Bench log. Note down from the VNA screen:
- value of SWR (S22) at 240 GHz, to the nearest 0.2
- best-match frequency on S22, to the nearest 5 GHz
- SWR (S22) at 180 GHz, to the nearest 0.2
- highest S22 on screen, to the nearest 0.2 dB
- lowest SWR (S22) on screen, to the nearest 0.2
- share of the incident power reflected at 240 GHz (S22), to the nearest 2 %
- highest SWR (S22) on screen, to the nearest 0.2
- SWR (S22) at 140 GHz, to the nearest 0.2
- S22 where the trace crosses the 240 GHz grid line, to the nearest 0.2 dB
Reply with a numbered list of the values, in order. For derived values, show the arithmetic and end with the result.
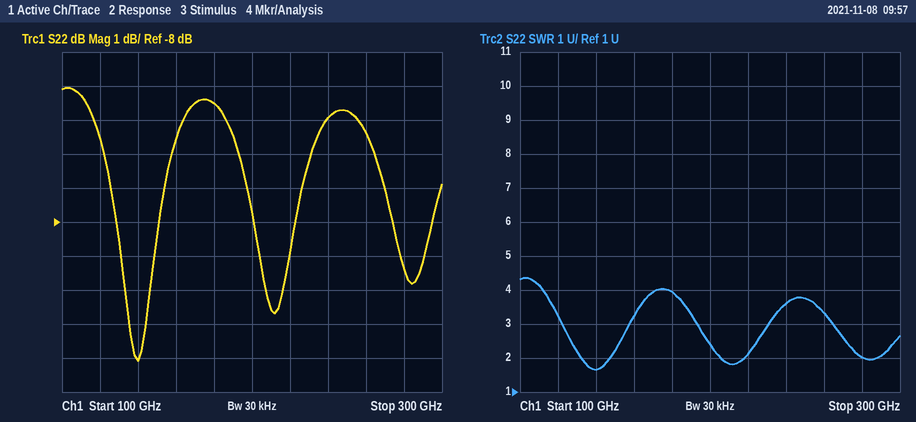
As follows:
1. 3.6
2. 140 GHz
3. 4.0
4. -4.0 dB
5. 1.6
6. 10^(-5/10) ≈ 32 %
7. 4.4
8. 1.6
9. -5.0 dB
